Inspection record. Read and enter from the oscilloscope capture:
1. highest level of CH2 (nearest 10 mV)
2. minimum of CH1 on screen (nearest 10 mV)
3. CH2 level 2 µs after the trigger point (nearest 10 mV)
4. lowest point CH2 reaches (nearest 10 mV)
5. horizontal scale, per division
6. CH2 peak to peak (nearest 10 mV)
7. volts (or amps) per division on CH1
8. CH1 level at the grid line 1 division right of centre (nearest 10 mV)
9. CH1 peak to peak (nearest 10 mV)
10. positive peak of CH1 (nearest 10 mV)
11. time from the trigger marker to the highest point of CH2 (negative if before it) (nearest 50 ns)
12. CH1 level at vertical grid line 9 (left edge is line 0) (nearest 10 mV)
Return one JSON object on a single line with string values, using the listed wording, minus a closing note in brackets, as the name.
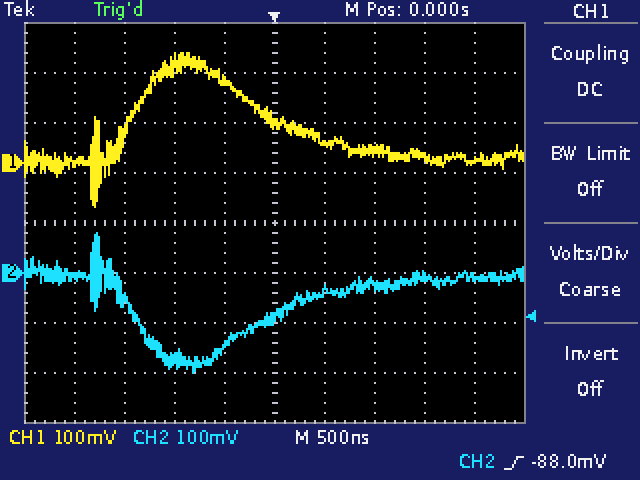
{"highest level of CH2": "80 mV", "minimum of CH1 on screen": "-90 mV", "CH2 level 2 µs after the trigger point": "-10 mV", "lowest point CH2 reaches": "-200 mV", "horizontal scale, per division": "500 ns", "CH2 peak to peak": "280 mV", "volts (or amps) per division on CH1": "100 mV", "CH1 level at the grid line 1 division right of centre": "40 mV", "CH1 peak to peak": "310 mV", "positive peak of CH1": "220 mV", "time from the trigger marker to the highest point of CH2 (negative if before it)": "-1.75 µs", "CH1 level at vertical grid line 9 (left edge is line 0)": "0 mV"}
